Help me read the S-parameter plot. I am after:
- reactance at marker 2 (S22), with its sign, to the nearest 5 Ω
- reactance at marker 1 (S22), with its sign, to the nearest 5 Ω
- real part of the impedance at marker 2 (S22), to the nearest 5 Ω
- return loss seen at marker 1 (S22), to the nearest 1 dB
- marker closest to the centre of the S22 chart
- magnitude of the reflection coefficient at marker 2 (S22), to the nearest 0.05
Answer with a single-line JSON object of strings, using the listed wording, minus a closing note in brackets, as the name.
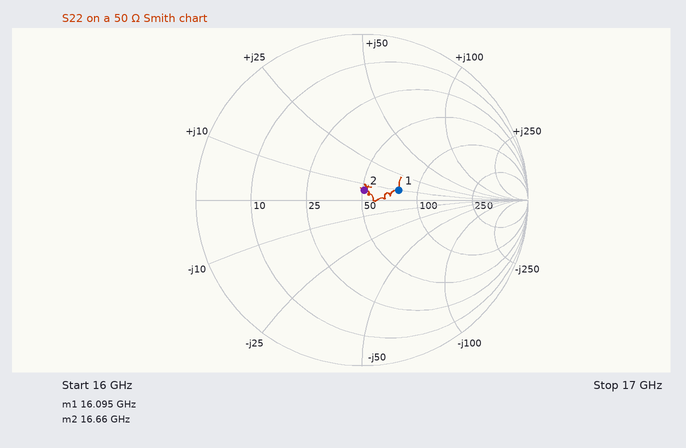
{"reactance at marker 2 (S22), with its sign, to the nearest 5 Ω": "+5 Ω", "reactance at marker 1 (S22), with its sign, to the nearest 5 Ω": "+10 Ω", "real part of the impedance at marker 2 (S22), to the nearest 5 Ω": "50 Ω", "return loss seen at marker 1 (S22), to the nearest 1 dB": "13 dB", "marker closest to the centre of the S22 chart": "marker 2", "magnitude of the reflection coefficient at marker 2 (S22), to the nearest 0.05": "0.05"}
